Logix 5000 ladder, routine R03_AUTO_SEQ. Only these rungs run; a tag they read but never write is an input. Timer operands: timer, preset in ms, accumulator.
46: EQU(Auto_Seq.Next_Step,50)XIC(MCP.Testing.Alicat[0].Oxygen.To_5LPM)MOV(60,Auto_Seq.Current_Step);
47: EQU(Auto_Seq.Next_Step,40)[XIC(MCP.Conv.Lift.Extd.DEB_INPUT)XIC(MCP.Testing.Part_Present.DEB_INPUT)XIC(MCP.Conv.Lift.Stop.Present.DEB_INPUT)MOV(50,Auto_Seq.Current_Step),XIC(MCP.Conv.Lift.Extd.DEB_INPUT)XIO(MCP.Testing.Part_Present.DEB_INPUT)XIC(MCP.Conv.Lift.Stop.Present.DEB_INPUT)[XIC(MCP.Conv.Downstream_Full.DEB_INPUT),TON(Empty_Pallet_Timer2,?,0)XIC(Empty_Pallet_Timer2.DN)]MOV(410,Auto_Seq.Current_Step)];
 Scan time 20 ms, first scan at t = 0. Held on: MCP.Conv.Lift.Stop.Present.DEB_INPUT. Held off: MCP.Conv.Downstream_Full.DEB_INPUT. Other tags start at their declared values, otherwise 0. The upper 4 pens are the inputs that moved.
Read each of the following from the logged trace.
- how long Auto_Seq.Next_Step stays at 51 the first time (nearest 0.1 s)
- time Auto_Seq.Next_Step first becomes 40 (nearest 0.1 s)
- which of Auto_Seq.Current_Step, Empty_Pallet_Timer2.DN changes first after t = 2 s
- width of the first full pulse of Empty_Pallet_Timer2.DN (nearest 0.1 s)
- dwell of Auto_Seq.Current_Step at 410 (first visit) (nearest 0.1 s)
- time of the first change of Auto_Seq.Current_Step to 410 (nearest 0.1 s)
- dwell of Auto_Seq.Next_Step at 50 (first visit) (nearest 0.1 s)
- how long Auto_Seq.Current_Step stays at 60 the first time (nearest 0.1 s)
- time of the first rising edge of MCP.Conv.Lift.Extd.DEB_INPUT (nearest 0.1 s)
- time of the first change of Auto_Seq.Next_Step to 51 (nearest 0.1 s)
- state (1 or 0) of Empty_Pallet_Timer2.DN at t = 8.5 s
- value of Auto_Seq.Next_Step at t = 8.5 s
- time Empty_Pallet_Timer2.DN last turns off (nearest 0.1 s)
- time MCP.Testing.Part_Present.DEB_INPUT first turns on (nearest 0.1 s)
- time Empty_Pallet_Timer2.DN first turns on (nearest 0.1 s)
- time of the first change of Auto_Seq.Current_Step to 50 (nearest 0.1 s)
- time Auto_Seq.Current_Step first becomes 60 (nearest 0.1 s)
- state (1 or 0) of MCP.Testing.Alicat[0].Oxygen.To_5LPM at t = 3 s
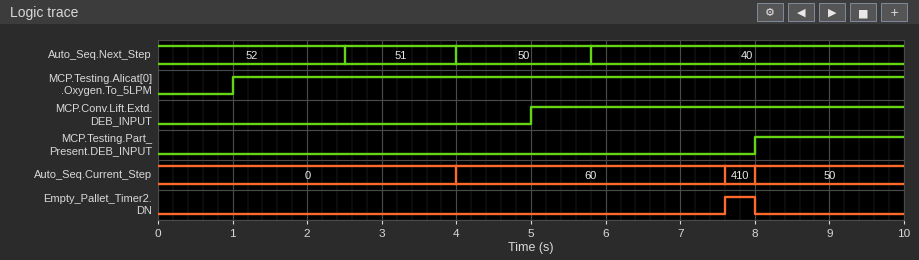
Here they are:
1.5 s
5.8 s
Auto_Seq.Current_Step
0.4 s
0.4 s
7.6 s
1.8 s
3.6 s
5.0 s
2.5 s
0
40
8.0 s
8.0 s
7.6 s
8.0 s
4.0 s
1
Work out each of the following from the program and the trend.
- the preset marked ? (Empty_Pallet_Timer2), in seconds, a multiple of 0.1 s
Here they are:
1.8 s
